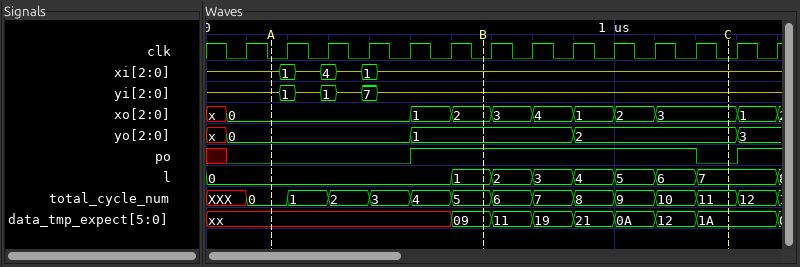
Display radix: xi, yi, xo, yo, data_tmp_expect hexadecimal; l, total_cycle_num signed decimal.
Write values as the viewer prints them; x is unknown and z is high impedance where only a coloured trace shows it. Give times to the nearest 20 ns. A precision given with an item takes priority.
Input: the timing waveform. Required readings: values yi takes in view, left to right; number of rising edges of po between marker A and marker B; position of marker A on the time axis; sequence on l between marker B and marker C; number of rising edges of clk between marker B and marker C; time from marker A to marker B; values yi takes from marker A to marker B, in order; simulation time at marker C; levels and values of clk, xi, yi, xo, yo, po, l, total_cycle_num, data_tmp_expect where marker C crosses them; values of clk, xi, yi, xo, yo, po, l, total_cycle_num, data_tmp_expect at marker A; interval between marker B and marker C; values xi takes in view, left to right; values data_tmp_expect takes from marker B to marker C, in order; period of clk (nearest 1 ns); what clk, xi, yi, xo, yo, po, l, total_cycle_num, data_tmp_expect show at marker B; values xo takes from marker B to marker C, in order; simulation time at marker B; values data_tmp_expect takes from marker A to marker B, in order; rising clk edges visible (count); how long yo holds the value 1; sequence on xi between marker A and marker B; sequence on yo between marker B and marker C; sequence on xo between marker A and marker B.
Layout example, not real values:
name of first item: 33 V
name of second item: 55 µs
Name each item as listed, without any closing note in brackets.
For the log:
values yi takes in view, left to right: z, 1, z, 1, z, 7, z
number of rising edges of po between marker A and marker B: 1
position of marker A on the time axis: 160 ns
sequence on l between marker B and marker C: 1, 2, 3, 4, 5, 6, 7
number of rising edges of clk between marker B and marker C: 6
time from marker A to marker B: 520 ns
values yi takes from marker A to marker B, in order: z, 1, z, 1, z, 7, z
simulation time at marker C: 1280 ns
levels and values of clk, xi, yi, xo, yo, po, l, total_cycle_num, data_tmp_expect where marker C crosses them: clk=0, xi=z, yi=z, xo=3, yo=2, po=0, l=7, total_cycle_num=11, data_tmp_expect=1A
values of clk, xi, yi, xo, yo, po, l, total_cycle_num, data_tmp_expect at marker A: clk=0, xi=z, yi=z, xo=0, yo=0, po=0, l=0, total_cycle_num=0, data_tmp_expect=xx
interval between marker B and marker C: 600 ns
values xi takes in view, left to right: z, 1, z, 4, z, 1, z
values data_tmp_expect takes from marker B to marker C, in order: 09, 11, 19, 21, 0A, 12, 1A
period of clk: 100 ns
what clk, xi, yi, xo, yo, po, l, total_cycle_num, data_tmp_expect show at marker B: clk=0, xi=z, yi=z, xo=2, yo=1, po=1, l=1, total_cycle_num=5, data_tmp_expect=09
values xo takes from marker B to marker C, in order: 2, 3, 4, 1, 2, 3
simulation time at marker B: 680 ns
values data_tmp_expect takes from marker A to marker B, in order: xx, 09
rising clk edges visible: 14
how long yo holds the value 1: 400 ns
sequence on xi between marker A and marker B: z, 1, z, 4, z, 1, z
sequence on yo between marker B and marker C: 1, 2
sequence on xo between marker A and marker B: 0, 1, 2
